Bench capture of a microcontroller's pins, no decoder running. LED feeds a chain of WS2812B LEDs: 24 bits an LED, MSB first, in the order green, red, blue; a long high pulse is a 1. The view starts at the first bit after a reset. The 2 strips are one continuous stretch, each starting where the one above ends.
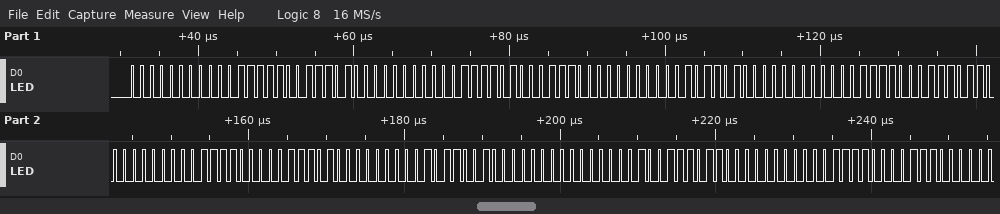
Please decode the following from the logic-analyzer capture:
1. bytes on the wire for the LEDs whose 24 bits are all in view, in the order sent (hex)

00 1F 3A 00 3D 1C 00 5A 00 1E 3B 00 3C 1D 00 59 00 01 3B 00 1E
